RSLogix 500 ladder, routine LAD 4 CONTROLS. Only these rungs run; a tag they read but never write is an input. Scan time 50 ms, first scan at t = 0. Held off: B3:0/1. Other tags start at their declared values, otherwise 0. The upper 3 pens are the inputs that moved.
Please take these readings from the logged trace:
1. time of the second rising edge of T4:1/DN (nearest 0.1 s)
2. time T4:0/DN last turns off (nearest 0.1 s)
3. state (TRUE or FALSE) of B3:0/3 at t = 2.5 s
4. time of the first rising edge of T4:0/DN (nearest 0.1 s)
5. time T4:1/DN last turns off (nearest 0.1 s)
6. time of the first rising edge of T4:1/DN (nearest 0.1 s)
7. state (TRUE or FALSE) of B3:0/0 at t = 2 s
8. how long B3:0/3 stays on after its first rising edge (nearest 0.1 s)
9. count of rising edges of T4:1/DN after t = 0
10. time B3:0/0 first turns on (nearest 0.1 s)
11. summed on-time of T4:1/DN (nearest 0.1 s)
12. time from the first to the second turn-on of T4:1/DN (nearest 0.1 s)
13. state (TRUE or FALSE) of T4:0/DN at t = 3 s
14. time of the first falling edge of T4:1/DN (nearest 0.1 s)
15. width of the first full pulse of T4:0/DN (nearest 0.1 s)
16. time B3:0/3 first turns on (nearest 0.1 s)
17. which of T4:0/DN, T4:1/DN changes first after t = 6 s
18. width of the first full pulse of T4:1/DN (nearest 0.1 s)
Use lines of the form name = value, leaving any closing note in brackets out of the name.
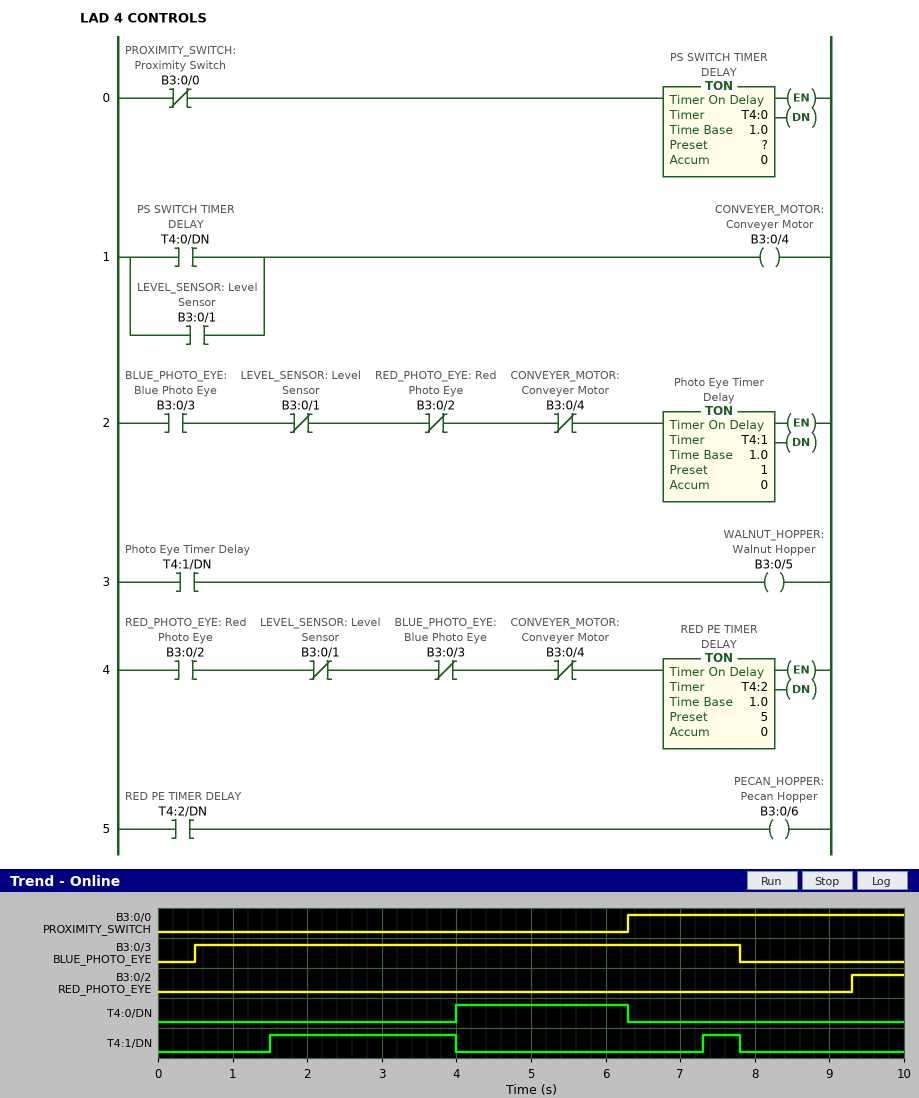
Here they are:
time of the second rising edge of T4:1/DN = 7.3 s
time T4:0/DN last turns off = 6.3 s
state (TRUE or FALSE) of B3:0/3 at t = 2.5 s = TRUE
time of the first rising edge of T4:0/DN = 4.0 s
time T4:1/DN last turns off = 7.8 s
time of the first rising edge of T4:1/DN = 1.5 s
state (TRUE or FALSE) of B3:0/0 at t = 2 s = FALSE
how long B3:0/3 stays on after its first rising edge = 7.3 s
count of rising edges of T4:1/DN after t = 0 = 2
time B3:0/0 first turns on = 6.3 s
summed on-time of T4:1/DN = 3.0 s
time from the first to the second turn-on of T4:1/DN = 5.8 s
state (TRUE or FALSE) of T4:0/DN at t = 3 s = FALSE
time of the first falling edge of T4:1/DN = 4.0 s
width of the first full pulse of T4:0/DN = 2.3 s
time B3:0/3 first turns on = 0.5 s
which of T4:0/DN, T4:1/DN changes first after t = 6 s = T4:0/DN
width of the first full pulse of T4:1/DN = 2.5 s
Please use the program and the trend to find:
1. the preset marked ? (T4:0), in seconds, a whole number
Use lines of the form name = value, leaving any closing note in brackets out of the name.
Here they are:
the preset marked ? (T4:0), in seconds, a whole number = 4 s
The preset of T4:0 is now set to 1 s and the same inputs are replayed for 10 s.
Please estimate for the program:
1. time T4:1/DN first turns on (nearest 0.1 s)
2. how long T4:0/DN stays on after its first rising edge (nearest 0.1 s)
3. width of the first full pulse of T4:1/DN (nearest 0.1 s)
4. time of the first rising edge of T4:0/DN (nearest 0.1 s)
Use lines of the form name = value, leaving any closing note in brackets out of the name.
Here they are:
time T4:1/DN first turns on = 7.3 s
how long T4:0/DN stays on after its first rising edge = 5.3 s
width of the first full pulse of T4:1/DN = 0.5 s
time of the first rising edge of T4:0/DN = 1.0 s
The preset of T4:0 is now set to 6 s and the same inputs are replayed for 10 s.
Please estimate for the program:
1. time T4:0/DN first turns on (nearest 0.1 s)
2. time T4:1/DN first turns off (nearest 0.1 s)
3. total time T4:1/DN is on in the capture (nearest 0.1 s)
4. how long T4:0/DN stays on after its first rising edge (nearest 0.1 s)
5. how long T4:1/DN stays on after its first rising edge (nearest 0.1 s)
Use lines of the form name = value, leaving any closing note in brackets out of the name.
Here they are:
time T4:0/DN first turns on = 6.0 s
time T4:1/DN first turns off = 6.0 s
total time T4:1/DN is on in the capture = 5.0 s
how long T4:0/DN stays on after its first rising edge = 0.3 s
how long T4:1/DN stays on after its first rising edge = 4.5 s
